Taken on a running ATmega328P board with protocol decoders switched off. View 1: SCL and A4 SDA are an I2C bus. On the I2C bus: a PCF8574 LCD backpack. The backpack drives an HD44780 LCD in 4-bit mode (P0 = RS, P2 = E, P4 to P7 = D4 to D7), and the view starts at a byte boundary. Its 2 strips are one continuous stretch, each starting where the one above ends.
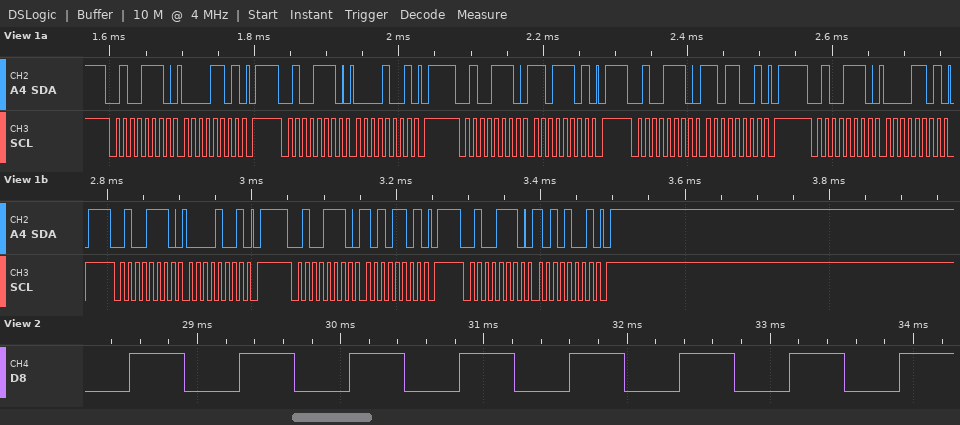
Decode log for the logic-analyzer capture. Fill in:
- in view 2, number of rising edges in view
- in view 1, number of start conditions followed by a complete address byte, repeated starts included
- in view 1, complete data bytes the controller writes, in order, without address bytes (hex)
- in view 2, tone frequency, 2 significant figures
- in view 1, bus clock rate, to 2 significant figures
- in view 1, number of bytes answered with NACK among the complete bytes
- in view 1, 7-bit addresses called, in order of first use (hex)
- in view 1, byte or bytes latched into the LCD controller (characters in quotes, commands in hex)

8
8
0D 09 DD D9 0D 09 AD A9
1.3 kHz
100 kHz
0
0x27
data 0x0D data 0x0A
